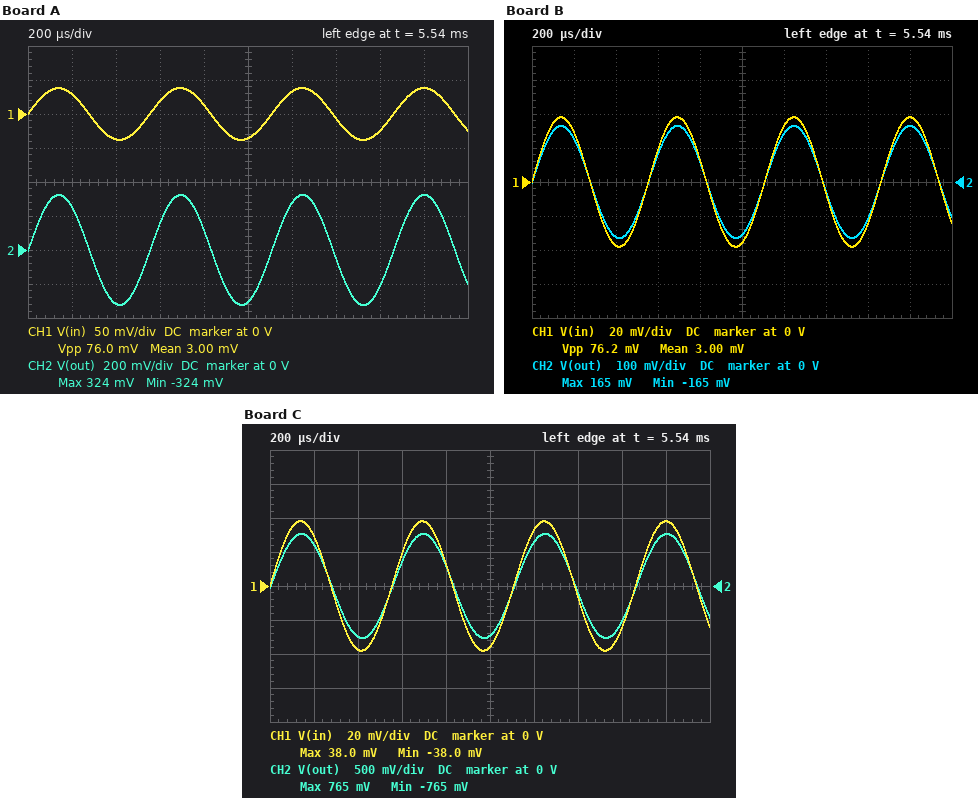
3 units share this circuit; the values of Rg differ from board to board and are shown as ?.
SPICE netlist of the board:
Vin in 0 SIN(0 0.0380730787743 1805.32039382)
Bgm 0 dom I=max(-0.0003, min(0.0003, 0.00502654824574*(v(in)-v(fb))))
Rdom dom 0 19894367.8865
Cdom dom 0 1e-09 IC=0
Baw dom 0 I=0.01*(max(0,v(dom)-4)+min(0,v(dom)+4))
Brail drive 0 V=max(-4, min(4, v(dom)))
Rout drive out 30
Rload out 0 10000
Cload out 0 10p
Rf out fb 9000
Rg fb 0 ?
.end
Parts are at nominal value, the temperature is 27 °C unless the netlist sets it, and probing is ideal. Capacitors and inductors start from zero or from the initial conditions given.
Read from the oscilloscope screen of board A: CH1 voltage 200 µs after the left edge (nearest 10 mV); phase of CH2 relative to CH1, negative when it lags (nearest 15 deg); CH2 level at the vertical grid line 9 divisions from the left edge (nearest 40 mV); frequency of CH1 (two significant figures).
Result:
30 mV
0 deg
320 mV
1.8 kHz
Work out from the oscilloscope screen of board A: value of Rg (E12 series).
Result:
1.2 kΩ
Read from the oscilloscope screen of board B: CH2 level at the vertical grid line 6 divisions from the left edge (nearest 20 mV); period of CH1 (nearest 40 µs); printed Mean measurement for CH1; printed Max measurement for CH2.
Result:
140 mV
560 µs
3.00 mV
165 mV
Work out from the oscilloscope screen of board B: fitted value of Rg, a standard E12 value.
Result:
2.7 kΩ
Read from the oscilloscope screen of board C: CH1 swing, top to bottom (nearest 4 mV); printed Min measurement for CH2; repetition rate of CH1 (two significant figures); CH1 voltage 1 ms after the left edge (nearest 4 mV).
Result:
76 mV
-765 mV
1.8 kHz
-36 mV
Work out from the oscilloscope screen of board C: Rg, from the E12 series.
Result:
470 Ω
